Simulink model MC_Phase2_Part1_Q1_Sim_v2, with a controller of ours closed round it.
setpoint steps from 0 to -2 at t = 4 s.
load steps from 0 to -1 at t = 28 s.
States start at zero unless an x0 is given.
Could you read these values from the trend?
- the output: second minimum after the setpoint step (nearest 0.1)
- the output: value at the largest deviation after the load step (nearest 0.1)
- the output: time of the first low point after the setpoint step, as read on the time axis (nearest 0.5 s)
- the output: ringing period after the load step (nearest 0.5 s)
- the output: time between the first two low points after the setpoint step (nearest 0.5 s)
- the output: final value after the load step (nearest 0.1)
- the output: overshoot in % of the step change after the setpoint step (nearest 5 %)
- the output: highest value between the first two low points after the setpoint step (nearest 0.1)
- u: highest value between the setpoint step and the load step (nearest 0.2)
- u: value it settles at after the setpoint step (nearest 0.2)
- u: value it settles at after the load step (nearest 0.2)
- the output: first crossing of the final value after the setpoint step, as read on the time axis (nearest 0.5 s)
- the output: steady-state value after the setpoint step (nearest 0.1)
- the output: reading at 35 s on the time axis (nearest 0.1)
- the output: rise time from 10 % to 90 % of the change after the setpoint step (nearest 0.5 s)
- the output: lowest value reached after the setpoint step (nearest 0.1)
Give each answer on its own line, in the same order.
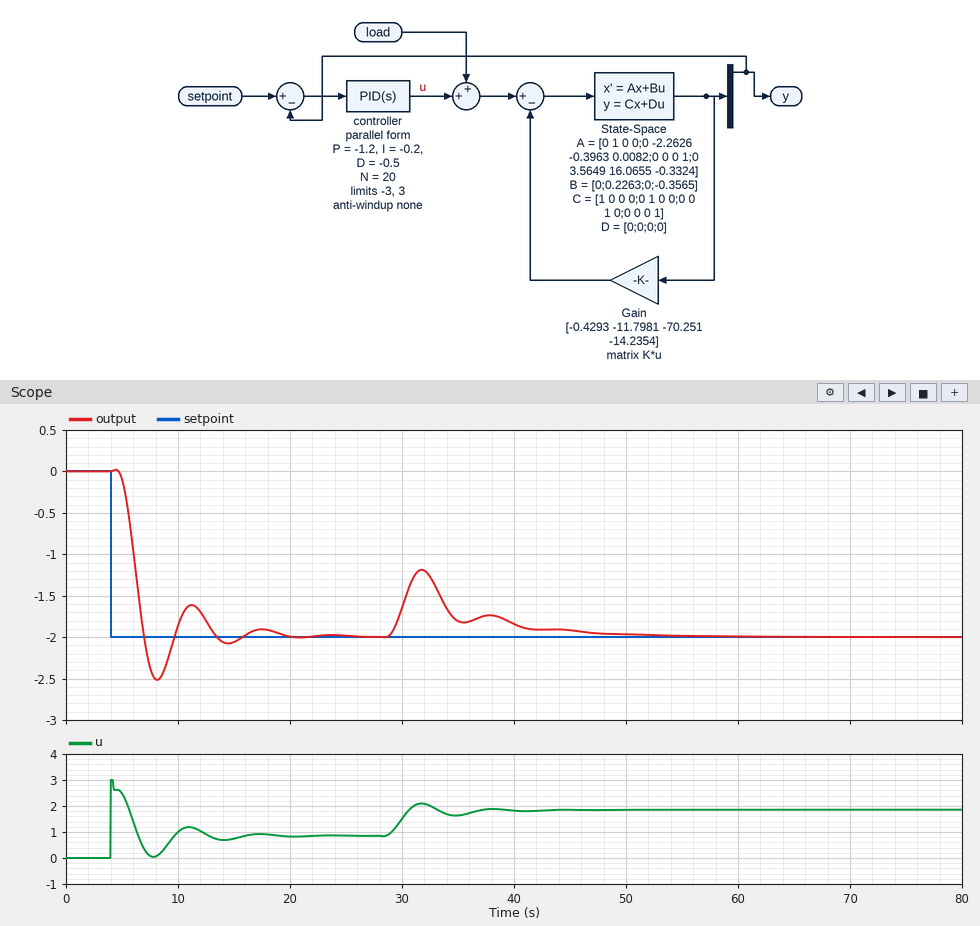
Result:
-2.1
-1.2
8.0 s
6.0 s
6.5 s
-2.0
25 %
-1.6
3.0
0.8
1.8
7.0 s
-2.0
-1.8
1.5 s
-2.5
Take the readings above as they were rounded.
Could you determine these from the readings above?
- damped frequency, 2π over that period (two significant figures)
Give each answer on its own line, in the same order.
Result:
0.97 rad/s
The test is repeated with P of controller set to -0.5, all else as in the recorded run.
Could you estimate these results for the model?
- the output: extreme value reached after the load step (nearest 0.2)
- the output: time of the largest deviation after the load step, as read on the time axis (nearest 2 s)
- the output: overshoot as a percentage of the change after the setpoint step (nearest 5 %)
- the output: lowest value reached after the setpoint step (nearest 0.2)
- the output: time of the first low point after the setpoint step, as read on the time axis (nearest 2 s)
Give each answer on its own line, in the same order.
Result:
-1.0
32 s
15 %
-2.2
12 s
